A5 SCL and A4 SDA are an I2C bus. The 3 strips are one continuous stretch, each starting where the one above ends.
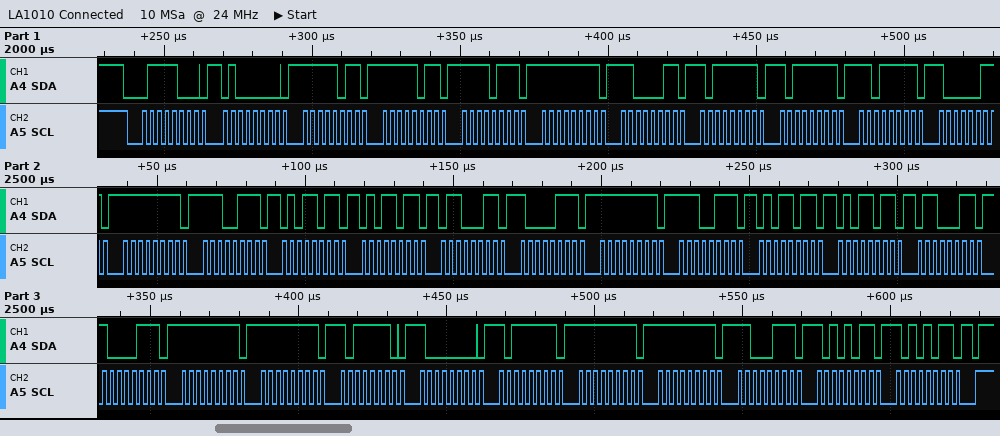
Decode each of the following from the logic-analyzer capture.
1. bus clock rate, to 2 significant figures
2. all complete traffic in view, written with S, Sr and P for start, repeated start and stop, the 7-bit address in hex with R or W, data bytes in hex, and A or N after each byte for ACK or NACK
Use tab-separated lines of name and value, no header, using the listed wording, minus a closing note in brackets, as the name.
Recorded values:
bus clock rate, to 2 significant figures	400 kHz
all complete traffic in view, written with S, Sr and P for start, repeated start and stop, the 7-bit address in hex with R or W, data bytes in hex, and A or N after each byte for ACK or NACK	S 3CW A 40 A FB A FB A F7 A FF A C3 A BF A BF A DF A 83 A FF A E7 A 5B A 5B A 63 A 87 A FF A E7 A 5B A 5B A 63 A 87 A FF A FF A BE A 80 A BF A FF A FF A C7 A AB A AB A P
